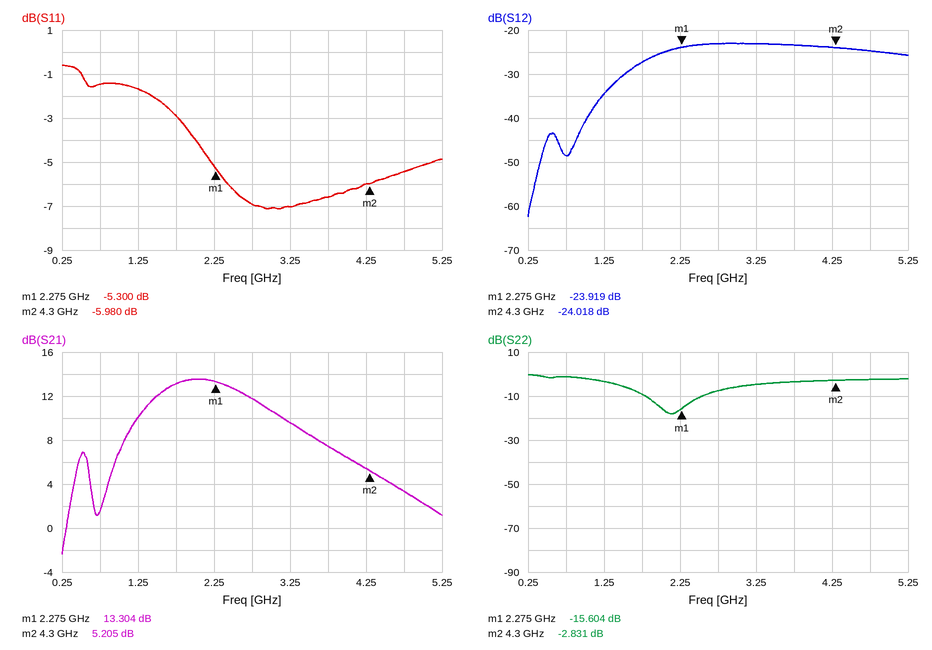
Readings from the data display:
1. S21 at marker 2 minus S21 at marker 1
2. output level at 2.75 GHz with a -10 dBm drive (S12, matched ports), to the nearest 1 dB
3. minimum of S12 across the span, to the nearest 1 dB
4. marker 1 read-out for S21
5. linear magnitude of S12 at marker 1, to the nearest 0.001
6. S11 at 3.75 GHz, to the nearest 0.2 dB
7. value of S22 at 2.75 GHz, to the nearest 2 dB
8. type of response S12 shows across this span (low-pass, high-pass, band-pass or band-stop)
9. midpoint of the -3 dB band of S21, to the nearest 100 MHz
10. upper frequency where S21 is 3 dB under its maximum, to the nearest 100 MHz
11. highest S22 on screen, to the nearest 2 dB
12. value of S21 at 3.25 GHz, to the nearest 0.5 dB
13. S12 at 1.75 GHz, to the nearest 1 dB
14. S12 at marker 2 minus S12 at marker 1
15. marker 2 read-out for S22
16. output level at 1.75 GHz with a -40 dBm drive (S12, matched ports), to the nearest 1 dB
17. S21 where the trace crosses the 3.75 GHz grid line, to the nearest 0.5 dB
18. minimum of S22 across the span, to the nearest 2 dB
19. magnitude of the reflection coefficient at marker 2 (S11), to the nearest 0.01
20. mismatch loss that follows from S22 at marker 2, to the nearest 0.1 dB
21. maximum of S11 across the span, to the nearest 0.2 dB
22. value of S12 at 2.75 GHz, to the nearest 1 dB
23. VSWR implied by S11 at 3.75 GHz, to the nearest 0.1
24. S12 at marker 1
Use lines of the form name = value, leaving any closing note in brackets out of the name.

S21 at marker 2 minus S21 at marker 1 = -8.099 dB
output level at 2.75 GHz with a -10 dBm drive (S12, matched ports), to the nearest 1 dB = -33 dBm
minimum of S12 across the span, to the nearest 1 dB = -62 dB
marker 1 read-out for S21 = 13.304 dB
linear magnitude of S12 at marker 1, to the nearest 0.001 = 0.064
S11 at 3.75 GHz, to the nearest 0.2 dB = -6.6 dB
value of S22 at 2.75 GHz, to the nearest 2 dB = -8 dB
type of response S12 shows across this span = high-pass
midpoint of the -3 dB band of S21, to the nearest 100 MHz = 2.2 GHz
upper frequency where S21 is 3 dB under its maximum, to the nearest 100 MHz = 3.0 GHz
highest S22 on screen, to the nearest 2 dB = 0 dB
value of S21 at 3.25 GHz, to the nearest 0.5 dB = 9.5 dB
S12 at 1.75 GHz, to the nearest 1 dB = -27 dB
S12 at marker 2 minus S12 at marker 1 = -0.099 dB
marker 2 read-out for S22 = -2.831 dB
output level at 1.75 GHz with a -40 dBm drive (S12, matched ports), to the nearest 1 dB = -67 dBm
S21 where the trace crosses the 3.75 GHz grid line, to the nearest 0.5 dB = 7.5 dB
minimum of S22 across the span, to the nearest 2 dB = -18 dB
magnitude of the reflection coefficient at marker 2 (S11), to the nearest 0.01 = 0.50
mismatch loss that follows from S22 at marker 2, to the nearest 0.1 dB = 3.2 dB
maximum of S11 across the span, to the nearest 0.2 dB = -0.6 dB
value of S12 at 2.75 GHz, to the nearest 1 dB = -23 dB
VSWR implied by S11 at 3.75 GHz, to the nearest 0.1 = 2.8
S12 at marker 1 = -23.919 dB
